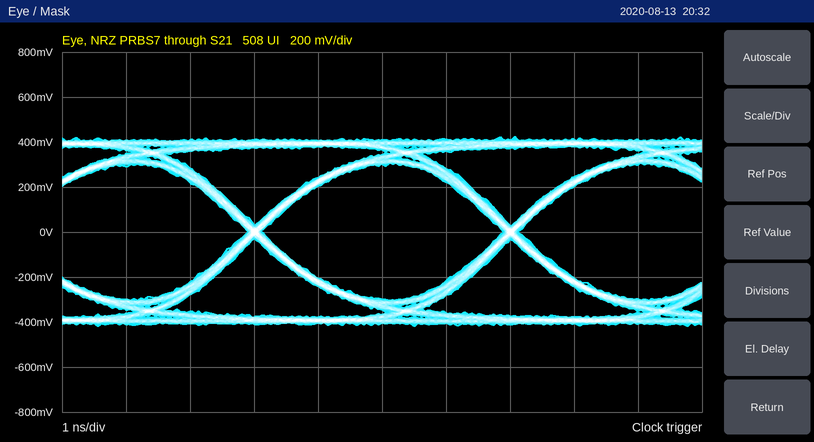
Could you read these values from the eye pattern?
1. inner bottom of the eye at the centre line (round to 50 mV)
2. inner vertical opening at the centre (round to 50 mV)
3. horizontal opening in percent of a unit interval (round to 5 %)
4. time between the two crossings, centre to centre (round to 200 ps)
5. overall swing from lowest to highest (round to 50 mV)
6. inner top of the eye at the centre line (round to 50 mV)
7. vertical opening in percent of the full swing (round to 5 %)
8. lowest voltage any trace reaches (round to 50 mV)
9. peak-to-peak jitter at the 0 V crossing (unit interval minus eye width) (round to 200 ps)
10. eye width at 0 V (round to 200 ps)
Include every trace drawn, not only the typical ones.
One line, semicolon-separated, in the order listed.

-300 mV; 600 mV; 95 %; 4.0 ns; 850 mV; 300 mV; 70 %; -400 mV; 200 ps; 3.8 ns
